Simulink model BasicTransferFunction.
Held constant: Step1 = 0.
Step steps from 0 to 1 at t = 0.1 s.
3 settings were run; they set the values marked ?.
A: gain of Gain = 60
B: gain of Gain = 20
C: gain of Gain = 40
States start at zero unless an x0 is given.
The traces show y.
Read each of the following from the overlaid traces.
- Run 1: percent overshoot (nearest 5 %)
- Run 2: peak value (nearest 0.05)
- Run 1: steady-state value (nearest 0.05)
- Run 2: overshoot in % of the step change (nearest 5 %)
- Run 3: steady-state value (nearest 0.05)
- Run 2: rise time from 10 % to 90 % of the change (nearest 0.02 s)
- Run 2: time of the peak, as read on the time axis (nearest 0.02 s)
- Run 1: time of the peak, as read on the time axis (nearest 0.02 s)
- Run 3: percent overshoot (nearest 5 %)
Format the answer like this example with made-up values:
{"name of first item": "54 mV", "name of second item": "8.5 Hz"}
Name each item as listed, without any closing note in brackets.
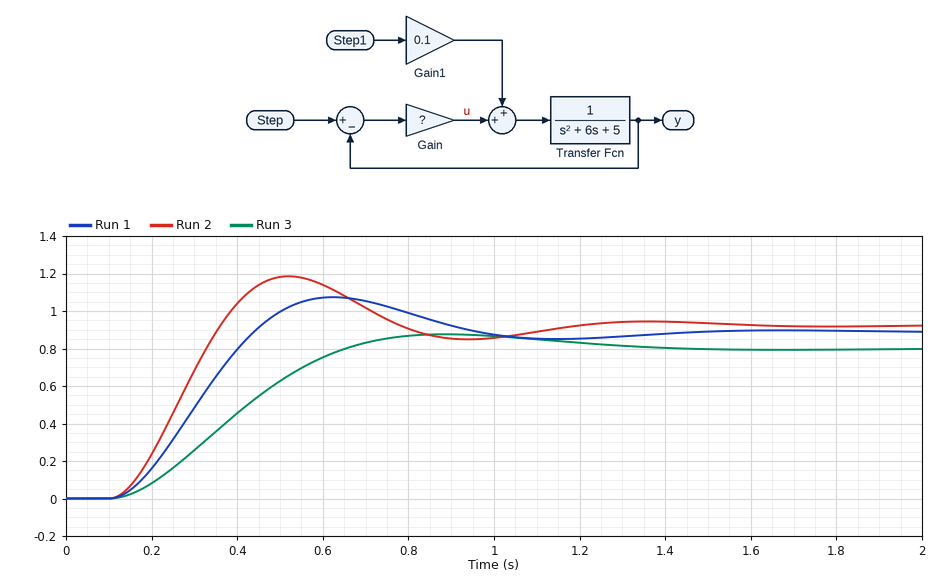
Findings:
{"Run 1: percent overshoot": "20 %", "Run 2: peak value": "1.20", "Run 1: steady-state value": "0.90", "Run 2: overshoot in % of the step change": "30 %", "Run 3: steady-state value": "0.80", "Run 2: rise time from 10 % to 90 % of the change": "0.18 s", "Run 2: time of the peak, as read on the time axis": "0.52 s", "Run 1: time of the peak, as read on the time axis": "0.62 s", "Run 3: percent overshoot": "10 %"}
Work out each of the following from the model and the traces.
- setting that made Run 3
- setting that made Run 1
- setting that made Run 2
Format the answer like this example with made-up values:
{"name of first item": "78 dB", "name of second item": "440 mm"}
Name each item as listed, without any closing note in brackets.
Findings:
{"setting that made Run 3": "B", "setting that made Run 1": "C", "setting that made Run 2": "A"}
